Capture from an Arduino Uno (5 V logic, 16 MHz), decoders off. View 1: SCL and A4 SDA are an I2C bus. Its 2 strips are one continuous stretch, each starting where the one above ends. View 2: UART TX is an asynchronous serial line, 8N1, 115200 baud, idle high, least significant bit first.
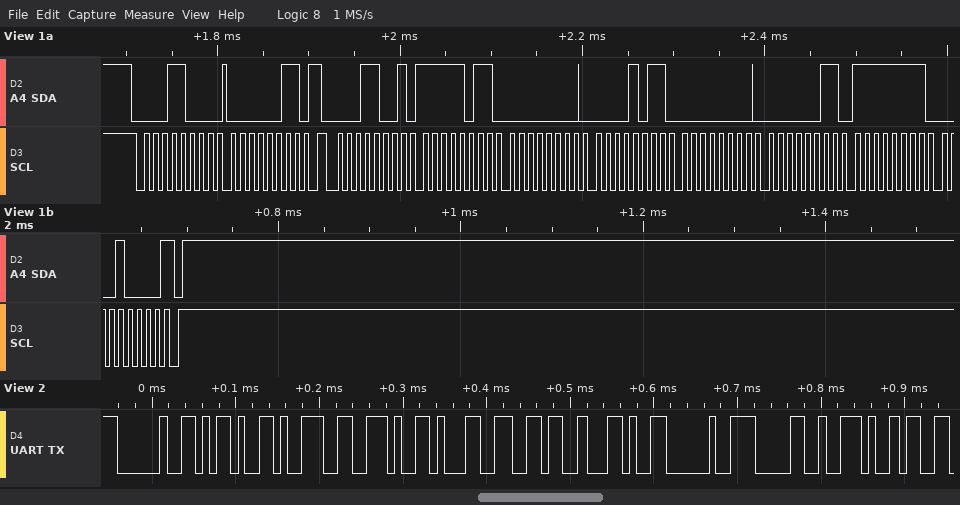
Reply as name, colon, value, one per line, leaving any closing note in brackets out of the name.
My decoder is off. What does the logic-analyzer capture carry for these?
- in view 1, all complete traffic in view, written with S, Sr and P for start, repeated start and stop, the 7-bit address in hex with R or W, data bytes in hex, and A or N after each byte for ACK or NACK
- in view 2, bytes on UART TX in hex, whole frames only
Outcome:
in view 1, all complete traffic in view, written with S, Sr and P for start, repeated start and stop, the 7-bit address in hex with R or W, data bytes in hex, and A or N after each byte for ACK or NACK: S 0CW A 03 A Sr 0CR A FB A 00 A 0B A 00 A 03 A FF A 10 N P
in view 2, bytes on UART TX in hex, whole frames only: 20 2D 39 2E 31 36 2C 20 30 2E
